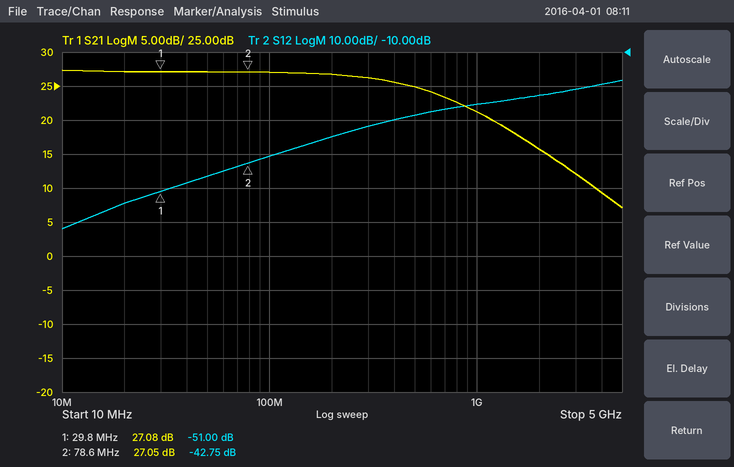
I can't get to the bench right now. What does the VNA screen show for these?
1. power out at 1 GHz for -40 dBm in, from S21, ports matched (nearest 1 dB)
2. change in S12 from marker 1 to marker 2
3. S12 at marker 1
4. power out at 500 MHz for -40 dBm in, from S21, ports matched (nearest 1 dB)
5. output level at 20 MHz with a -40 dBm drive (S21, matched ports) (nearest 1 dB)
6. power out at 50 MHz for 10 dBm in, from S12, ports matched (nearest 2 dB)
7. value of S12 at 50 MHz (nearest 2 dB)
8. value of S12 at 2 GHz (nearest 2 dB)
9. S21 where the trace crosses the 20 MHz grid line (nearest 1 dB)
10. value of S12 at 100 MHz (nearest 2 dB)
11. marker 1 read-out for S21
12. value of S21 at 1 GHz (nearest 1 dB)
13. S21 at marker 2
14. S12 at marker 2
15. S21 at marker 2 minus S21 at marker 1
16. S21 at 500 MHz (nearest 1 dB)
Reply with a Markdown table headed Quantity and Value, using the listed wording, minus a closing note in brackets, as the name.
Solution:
| Quantity | Value |
|---|---|
| power out at 1 GHz for -40 dBm in, from S21, ports matched | -19 dBm |
| change in S12 from marker 1 to marker 2 | 8.25 dB |
| S12 at marker 1 | -51.00 dB |
| power out at 500 MHz for -40 dBm in, from S21, ports matched | -15 dBm |
| output level at 20 MHz with a -40 dBm drive (S21, matched ports) | -13 dBm |
| power out at 50 MHz for 10 dBm in, from S12, ports matched | -36 dBm |
| value of S12 at 50 MHz | -46 dB |
| value of S12 at 2 GHz | -22 dB |
| S21 where the trace crosses the 20 MHz grid line | 27 dB |
| value of S12 at 100 MHz | -40 dB |
| marker 1 read-out for S21 | 27.08 dB |
| value of S21 at 1 GHz | 21 dB |
| S21 at marker 2 | 27.05 dB |
| S12 at marker 2 | -42.75 dB |
| S21 at marker 2 minus S21 at marker 1 | -0.03 dB |
| S21 at 500 MHz | 25 dB |
